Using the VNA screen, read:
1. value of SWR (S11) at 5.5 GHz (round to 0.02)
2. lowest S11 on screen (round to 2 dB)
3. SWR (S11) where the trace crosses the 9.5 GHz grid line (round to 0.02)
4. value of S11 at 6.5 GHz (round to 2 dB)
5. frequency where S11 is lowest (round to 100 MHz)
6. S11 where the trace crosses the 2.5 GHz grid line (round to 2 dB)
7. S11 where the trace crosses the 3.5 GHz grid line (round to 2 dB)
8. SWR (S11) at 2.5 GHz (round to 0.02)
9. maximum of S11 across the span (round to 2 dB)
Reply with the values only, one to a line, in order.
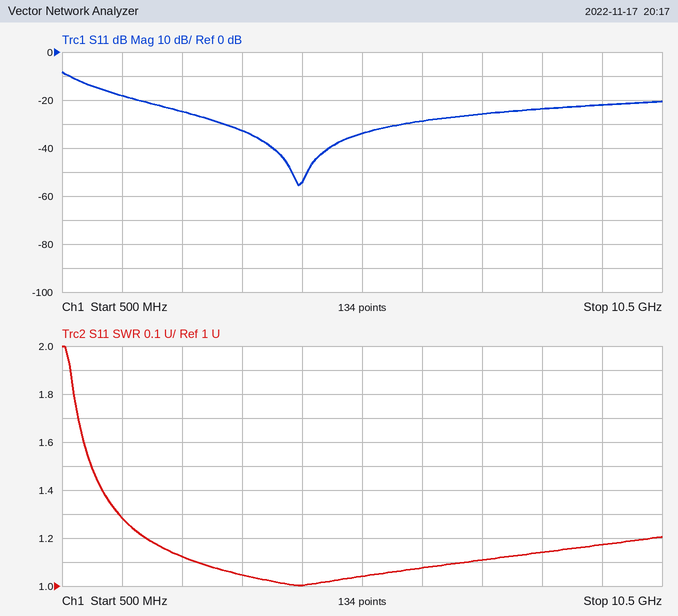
1.04
-56 dB
1.18
-28 dB
4.4 GHz
-24 dB
-32 dB
1.12
-8 dB
